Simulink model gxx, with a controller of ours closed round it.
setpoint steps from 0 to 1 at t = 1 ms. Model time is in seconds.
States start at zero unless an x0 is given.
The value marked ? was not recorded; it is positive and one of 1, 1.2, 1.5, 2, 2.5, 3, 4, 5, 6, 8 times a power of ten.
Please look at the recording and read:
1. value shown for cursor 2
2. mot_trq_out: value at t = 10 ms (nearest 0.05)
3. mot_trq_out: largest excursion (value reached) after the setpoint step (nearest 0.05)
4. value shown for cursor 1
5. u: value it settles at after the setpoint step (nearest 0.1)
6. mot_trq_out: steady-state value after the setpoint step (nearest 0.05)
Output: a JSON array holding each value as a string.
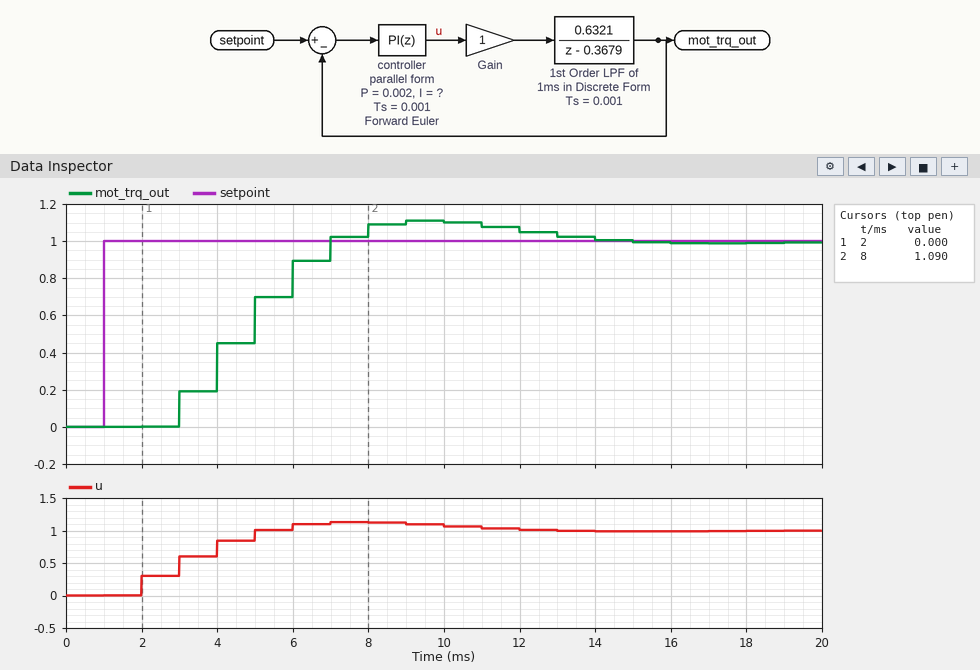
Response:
["1.090", "1.10", "1.10", "0.000", "1.0", "1.00"]
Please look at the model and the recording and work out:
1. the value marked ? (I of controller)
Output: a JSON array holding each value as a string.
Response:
["300"]
